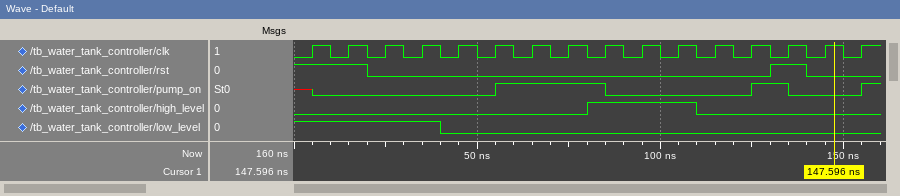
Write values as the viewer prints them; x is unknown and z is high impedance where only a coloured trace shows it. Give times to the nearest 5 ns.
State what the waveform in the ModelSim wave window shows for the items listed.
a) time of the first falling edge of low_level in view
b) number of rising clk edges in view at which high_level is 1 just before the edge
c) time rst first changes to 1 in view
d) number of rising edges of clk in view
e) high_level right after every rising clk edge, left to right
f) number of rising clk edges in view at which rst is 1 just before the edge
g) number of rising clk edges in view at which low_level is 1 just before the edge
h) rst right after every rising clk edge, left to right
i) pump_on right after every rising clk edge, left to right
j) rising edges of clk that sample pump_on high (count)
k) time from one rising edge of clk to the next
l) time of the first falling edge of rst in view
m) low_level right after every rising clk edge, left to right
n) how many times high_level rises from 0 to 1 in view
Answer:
40 ns
3
130 ns
16
0 0 0 0 0 0 0 0 1 1 1 0 0 0 0 0
3
4
1 1 0 0 0 0 0 0 0 0 0 0 0 1 0 0
0 0 0 0 0 1 1 1 0 0 0 0 1 0 0 1
4
10 ns
20 ns
1 1 1 1 0 0 0 0 0 0 0 0 0 0 0 0
1
